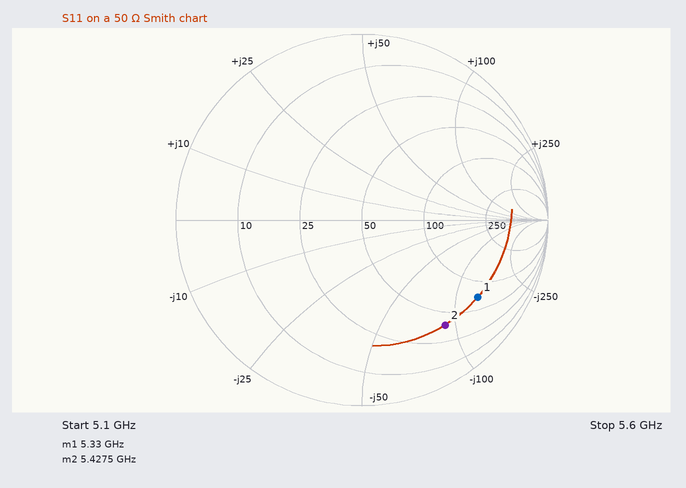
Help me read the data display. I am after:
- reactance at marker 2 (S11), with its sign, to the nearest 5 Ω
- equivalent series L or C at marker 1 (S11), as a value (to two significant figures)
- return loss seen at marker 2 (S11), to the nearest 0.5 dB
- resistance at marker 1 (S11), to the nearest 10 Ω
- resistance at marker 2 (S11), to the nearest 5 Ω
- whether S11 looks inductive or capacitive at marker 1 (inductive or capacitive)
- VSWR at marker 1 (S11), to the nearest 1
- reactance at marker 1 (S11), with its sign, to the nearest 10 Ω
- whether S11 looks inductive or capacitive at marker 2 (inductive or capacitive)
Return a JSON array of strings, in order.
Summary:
["-90 Ω", "230 fF", "3.0 dB", "70 Ω", "40 Ω", "capacitive", "7", "-130 Ω", "capacitive"]
